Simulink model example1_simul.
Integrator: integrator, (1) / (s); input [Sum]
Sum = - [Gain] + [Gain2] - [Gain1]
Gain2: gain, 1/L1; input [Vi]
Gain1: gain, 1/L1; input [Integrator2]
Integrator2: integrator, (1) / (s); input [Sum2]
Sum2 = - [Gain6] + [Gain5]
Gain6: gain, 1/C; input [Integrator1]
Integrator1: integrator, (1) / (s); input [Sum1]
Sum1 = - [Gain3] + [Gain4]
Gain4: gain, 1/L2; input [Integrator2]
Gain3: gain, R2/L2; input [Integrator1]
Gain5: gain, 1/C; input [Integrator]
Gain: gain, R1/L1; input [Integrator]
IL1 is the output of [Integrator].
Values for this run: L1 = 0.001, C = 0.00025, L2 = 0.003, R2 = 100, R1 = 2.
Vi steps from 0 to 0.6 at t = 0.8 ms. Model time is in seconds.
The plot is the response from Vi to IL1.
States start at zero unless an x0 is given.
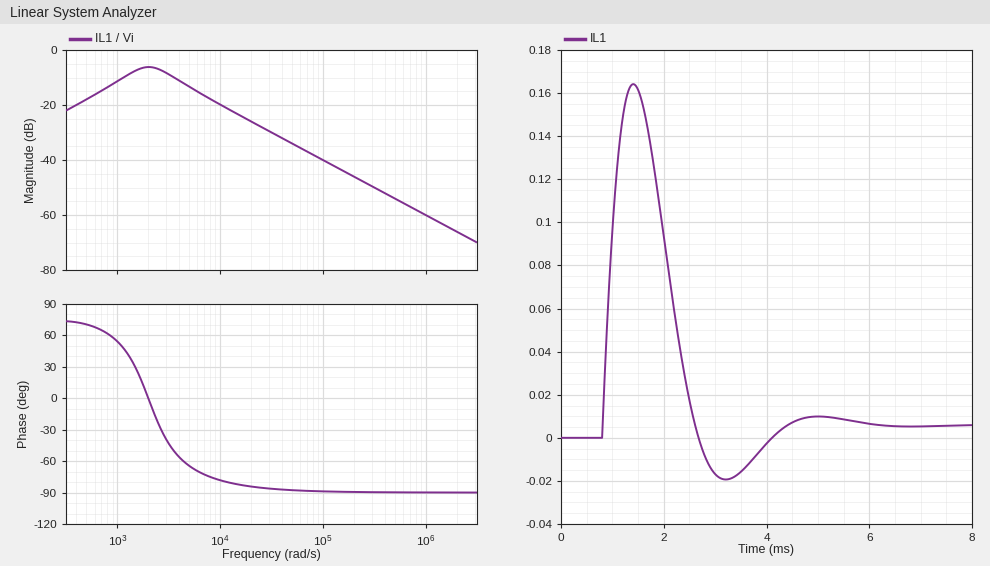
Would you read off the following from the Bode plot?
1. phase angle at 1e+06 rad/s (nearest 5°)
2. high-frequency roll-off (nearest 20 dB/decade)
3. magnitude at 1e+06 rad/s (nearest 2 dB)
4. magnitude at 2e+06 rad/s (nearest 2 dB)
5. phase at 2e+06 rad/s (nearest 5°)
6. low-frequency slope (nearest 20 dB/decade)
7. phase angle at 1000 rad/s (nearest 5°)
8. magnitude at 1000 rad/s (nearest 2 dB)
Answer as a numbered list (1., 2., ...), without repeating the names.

1. -90°
2. -20 dB/decade
3. -60 dB
4. -66 dB
5. -90°
6. 20 dB/decade
7. 55°
8. -12 dB
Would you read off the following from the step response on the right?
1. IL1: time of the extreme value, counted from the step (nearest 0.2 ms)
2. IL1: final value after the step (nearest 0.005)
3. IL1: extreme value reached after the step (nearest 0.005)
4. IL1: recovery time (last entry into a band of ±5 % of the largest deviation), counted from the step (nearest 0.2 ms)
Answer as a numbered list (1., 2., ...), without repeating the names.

1. 0.6 ms
2. 0.005
3. 0.165
4. 3.2 ms
